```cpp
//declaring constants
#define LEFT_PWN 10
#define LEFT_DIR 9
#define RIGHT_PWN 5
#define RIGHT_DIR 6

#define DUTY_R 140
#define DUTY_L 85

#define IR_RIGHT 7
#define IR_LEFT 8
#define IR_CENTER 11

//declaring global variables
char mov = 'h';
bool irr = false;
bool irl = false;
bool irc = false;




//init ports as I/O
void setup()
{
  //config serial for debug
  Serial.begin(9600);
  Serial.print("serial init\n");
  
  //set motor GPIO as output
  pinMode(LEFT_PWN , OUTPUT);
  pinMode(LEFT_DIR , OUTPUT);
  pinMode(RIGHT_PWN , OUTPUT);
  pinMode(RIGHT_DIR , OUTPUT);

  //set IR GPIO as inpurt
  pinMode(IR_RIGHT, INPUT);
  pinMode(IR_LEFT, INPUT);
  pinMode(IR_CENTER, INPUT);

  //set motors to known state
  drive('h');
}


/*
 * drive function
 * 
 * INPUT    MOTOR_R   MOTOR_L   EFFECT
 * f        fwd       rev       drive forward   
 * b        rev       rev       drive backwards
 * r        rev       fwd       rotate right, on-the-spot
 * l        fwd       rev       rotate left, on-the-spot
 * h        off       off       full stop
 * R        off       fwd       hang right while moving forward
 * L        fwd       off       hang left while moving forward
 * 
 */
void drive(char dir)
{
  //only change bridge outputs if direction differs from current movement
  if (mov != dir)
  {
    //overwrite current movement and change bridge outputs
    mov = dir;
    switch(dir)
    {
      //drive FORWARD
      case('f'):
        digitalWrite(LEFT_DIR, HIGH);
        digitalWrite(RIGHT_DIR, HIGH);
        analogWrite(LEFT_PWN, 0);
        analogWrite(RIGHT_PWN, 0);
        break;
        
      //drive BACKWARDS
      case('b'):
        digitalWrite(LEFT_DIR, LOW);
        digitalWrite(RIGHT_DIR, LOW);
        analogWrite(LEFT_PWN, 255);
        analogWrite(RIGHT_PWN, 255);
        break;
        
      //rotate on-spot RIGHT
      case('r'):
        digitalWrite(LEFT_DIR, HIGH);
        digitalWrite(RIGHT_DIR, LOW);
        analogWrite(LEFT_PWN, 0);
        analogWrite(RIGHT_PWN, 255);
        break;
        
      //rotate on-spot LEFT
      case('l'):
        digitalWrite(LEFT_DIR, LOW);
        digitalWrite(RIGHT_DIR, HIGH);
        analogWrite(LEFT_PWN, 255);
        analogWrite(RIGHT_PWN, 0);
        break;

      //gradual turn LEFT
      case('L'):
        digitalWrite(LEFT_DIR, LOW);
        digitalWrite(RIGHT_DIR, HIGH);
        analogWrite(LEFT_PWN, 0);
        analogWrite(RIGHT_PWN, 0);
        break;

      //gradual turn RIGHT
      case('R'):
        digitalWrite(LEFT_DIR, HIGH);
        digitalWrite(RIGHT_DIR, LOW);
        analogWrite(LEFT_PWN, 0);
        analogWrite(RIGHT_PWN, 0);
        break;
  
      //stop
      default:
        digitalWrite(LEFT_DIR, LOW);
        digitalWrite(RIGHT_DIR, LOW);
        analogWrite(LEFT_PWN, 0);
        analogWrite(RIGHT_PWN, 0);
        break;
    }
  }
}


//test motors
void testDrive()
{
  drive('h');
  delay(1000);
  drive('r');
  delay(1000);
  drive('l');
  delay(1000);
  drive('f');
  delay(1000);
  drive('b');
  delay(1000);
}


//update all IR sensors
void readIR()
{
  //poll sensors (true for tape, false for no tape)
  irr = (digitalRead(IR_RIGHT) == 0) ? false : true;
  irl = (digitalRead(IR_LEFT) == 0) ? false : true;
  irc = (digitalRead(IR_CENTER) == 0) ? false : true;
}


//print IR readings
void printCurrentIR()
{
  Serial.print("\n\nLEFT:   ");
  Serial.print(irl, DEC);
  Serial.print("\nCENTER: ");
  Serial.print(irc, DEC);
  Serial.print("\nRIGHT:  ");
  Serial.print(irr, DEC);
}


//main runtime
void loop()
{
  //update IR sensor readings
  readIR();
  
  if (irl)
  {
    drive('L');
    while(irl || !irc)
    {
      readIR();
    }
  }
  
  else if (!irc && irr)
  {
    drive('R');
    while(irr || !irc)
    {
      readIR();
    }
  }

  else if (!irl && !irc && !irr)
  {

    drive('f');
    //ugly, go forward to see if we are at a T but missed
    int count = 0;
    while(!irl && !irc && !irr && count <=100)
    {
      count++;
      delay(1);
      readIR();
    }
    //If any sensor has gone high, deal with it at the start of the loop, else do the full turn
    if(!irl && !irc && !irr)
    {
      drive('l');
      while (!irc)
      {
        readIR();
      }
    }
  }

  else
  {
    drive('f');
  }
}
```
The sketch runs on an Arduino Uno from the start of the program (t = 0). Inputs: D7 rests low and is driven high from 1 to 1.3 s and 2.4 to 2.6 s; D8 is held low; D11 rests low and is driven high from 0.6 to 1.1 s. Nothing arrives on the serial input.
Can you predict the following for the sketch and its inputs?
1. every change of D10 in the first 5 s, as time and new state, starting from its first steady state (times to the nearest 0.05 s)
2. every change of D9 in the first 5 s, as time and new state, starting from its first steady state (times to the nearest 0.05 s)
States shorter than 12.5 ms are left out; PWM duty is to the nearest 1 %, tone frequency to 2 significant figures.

0 s low; 0.1 s high; 0.6 s low
0 s high; 0.1 s low; 0.6 s high
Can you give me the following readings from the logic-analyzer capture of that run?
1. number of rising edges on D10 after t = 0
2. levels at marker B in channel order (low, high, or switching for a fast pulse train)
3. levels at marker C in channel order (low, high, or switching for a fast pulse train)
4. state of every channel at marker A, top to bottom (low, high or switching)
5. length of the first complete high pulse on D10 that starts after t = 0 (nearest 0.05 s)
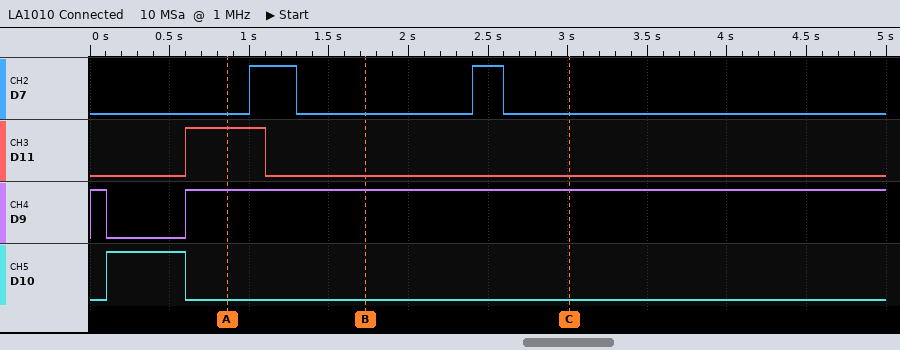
1
D7 low, D11 low, D9 high, D10 low
D7 low, D11 low, D9 high, D10 low
D7 low, D11 high, D9 high, D10 low
0.50 s
